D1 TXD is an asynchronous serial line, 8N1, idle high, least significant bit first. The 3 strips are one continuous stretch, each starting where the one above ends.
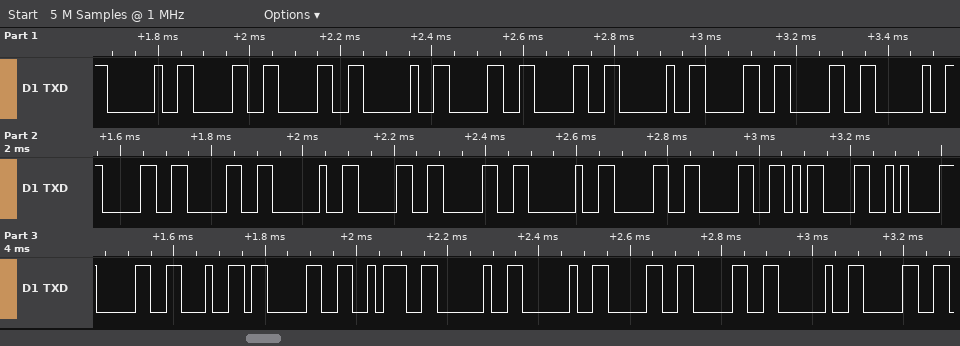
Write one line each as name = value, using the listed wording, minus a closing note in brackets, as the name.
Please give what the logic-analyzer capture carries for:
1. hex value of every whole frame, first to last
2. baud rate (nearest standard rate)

hex value of every whole frame, first to last = 20 30 30 20 30 30 20 30 30 20 30 30 20 30 30 20 30 30 0D 0A 30 64 30 3A 20 20 30 30 20 30
baud rate = 57600 baud
